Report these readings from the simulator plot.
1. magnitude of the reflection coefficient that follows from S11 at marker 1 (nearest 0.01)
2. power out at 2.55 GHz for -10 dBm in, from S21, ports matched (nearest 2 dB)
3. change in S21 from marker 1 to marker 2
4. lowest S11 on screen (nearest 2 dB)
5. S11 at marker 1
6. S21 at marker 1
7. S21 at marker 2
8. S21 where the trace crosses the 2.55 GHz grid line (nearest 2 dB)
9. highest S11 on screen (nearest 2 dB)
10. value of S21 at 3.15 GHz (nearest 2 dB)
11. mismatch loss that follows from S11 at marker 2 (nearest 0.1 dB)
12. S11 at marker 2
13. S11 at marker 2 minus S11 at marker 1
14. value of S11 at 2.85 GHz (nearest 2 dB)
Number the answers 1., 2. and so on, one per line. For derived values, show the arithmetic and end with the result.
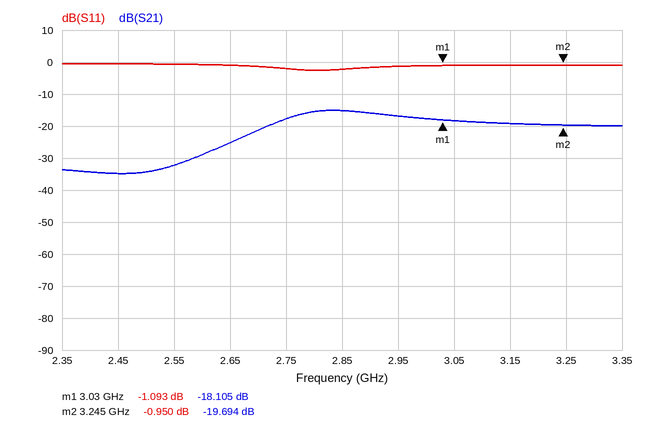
1. 10^(-1.093/20) ≈ 0.88
2. -10 dBm + (-32 dB) = -42 dBm
3. -19.694 − (-18.105) = -1.589 dB
4. -2 dB
5. -1.093 dB
6. -18.105 dB
7. -19.694 dB
8. -32 dB
9. 0 dB
10. -20 dB
11. −10 log10(1 − 10^(-0.95/10)) ≈ 7.1 dB
12. -0.950 dB
13. -0.95 − (-1.093) = 0.143 dB
14. -2 dB
